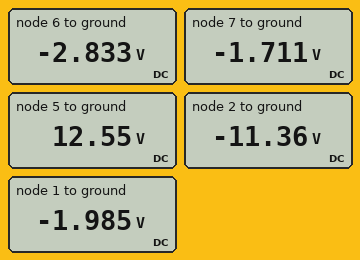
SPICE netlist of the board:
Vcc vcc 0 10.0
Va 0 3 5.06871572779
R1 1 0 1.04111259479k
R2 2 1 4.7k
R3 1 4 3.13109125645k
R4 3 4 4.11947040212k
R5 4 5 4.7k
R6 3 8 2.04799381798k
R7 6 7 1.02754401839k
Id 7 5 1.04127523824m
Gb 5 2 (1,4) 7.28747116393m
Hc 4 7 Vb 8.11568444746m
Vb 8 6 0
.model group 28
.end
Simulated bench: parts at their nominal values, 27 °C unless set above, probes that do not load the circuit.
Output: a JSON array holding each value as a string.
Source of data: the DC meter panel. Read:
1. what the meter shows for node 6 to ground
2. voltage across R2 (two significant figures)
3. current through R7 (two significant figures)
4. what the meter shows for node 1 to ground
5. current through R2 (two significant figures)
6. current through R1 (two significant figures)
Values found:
["-2.833 V", "9.4 V", "1.1 mA", "-1.985 V", "2.0 mA", "1.9 mA"]
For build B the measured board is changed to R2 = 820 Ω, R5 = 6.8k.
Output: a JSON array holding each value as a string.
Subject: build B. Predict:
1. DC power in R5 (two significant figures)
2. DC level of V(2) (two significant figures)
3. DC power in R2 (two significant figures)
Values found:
["63 mW", "-3.6 V", "3.3 mW"]
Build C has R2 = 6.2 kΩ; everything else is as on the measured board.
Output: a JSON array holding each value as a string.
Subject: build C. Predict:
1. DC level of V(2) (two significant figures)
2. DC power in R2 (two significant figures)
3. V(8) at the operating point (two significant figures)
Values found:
["-14 V", "25 mW", "-2.8 V"]
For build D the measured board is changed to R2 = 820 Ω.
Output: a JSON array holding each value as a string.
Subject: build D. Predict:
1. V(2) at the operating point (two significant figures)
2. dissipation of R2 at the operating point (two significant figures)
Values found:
["-3.6 V", "3.3 mW"]
